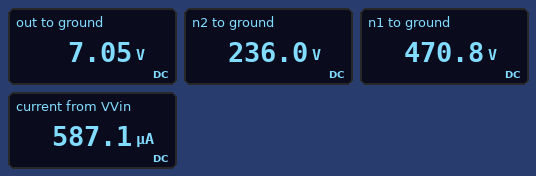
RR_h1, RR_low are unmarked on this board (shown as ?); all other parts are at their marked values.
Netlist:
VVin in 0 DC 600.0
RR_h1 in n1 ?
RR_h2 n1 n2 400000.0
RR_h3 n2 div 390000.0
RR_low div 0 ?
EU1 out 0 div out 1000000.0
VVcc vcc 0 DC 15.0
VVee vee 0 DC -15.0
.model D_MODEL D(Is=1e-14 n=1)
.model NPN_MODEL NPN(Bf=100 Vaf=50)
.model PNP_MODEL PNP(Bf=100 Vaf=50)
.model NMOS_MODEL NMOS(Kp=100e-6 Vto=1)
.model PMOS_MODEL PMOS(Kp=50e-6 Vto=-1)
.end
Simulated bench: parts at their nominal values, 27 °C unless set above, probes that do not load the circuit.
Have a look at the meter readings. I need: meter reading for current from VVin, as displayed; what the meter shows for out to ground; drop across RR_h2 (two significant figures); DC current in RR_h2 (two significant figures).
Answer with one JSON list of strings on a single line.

["587.1 µA", "7.05 V", "230 V", "590 µA"]
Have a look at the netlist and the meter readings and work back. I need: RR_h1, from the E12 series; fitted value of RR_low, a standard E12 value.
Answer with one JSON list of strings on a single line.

["220 kΩ", "12 kΩ"]
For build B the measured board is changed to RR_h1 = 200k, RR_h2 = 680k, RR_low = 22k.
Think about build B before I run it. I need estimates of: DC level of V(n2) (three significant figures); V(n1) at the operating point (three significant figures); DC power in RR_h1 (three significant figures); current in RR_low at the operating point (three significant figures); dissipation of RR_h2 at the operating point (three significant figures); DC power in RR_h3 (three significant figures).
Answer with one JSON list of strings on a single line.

["191 V", "507 V", "43.1 mW", "464 µA", "147 mW", "84.1 mW"]
